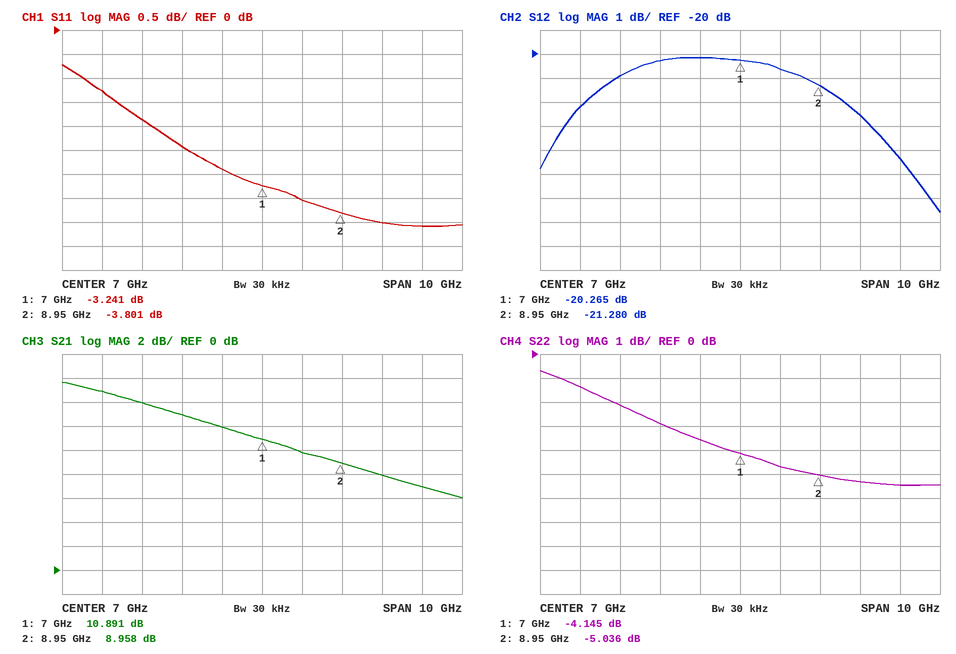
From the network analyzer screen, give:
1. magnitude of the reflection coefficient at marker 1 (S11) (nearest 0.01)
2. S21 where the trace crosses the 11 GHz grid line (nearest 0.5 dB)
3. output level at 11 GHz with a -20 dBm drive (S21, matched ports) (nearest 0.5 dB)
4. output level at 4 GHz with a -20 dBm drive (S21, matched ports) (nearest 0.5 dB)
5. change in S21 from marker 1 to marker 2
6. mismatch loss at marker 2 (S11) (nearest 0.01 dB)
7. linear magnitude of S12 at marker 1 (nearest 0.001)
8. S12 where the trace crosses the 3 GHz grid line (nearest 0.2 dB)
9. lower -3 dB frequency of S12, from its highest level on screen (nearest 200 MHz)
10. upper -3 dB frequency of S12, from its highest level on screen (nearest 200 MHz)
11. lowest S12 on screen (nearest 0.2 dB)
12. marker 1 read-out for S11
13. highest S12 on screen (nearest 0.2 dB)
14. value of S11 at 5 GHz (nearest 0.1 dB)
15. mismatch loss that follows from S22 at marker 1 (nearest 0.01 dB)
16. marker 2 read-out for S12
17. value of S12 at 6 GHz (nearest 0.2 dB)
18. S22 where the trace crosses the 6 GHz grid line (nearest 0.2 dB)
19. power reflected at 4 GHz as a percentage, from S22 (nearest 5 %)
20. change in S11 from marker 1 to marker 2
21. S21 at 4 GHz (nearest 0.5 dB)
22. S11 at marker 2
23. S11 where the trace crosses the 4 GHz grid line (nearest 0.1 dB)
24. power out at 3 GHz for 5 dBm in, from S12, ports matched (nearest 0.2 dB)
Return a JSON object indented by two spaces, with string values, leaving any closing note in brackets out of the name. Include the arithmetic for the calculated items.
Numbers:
{
  "magnitude of the reflection coefficient at marker 1 (S11)": "10^(-3.241/20) ≈ 0.69",
  "S21 where the trace crosses the 11 GHz grid line": "7.0 dB",
  "output level at 11 GHz with a -20 dBm drive (S21, matched ports)": "-20 dBm + (7.0 dB) = -13.0 dBm",
  "output level at 4 GHz with a -20 dBm drive (S21, matched ports)": "-20 dBm + (14.0 dB) = -6.0 dBm",
  "change in S21 from marker 1 to marker 2": "8.958 − (10.891) = -1.933 dB",
  "mismatch loss at marker 2 (S11)": "−10 log10(1 − 10^(-3.801/10)) ≈ 2.34 dB",
  "linear magnitude of S12 at marker 1": "10^(-20.265/20) ≈ 0.097",
  "S12 where the trace crosses the 3 GHz grid line": "-22.2 dB",
  "lower -3 dB frequency of S12, from its highest level on screen": "2.6 GHz",
  "upper -3 dB frequency of S12, from its highest level on screen": "10.4 GHz",
  "lowest S12 on screen": "-26.6 dB",
  "marker 1 read-out for S11": "-3.241 dB",
  "highest S12 on screen": "-20.2 dB",
  "value of S11 at 5 GHz": "-2.4 dB",
  "mismatch loss that follows from S22 at marker 1": "−10 log10(1 − 10^(-4.145/10)) ≈ 2.11 dB",
  "marker 2 read-out for S12": "-21.280 dB",
  "value of S12 at 6 GHz": "-20.2 dB",
  "S22 where the trace crosses the 6 GHz grid line": "-3.6 dB",
  "power reflected at 4 GHz as a percentage, from S22": "10^(-2.2/10) ≈ 60 %",
  "change in S11 from marker 1 to marker 2": "-3.801 − (-3.241) = -0.560 dB",
  "S21 at 4 GHz": "14.0 dB",
  "S11 at marker 2": "-3.801 dB",
  "S11 where the trace crosses the 4 GHz grid line": "-1.9 dB",
  "power out at 3 GHz for 5 dBm in, from S12, ports matched": "5 dBm + (-22.2 dB) = -17.2 dBm"
}
